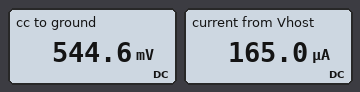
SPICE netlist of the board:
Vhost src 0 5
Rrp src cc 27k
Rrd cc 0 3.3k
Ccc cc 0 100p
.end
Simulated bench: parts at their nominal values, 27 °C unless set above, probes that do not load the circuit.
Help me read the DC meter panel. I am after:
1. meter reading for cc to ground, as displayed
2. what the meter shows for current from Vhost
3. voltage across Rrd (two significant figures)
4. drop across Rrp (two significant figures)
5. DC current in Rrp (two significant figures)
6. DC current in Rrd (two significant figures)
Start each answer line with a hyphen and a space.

- 544.6 mV
- 165.0 µA
- 540 mV
- 4.5 V
- 170 µA
- 170 µA
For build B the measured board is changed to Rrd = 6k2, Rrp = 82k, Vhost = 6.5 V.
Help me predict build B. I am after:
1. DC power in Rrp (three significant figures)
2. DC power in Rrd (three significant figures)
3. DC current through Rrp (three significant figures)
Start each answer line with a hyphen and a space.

- 445 µW
- 33.7 µW
- 73.7 µA
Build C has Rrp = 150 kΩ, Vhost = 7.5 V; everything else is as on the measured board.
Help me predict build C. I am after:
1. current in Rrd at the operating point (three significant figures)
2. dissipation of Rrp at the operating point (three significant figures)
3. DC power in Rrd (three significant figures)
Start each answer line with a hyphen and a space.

- 48.9 µA
- 359 µW
- 7.90 µW
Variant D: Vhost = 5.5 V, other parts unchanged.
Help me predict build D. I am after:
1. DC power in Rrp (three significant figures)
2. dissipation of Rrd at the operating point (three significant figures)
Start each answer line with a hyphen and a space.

- 890 µW
- 109 µW
